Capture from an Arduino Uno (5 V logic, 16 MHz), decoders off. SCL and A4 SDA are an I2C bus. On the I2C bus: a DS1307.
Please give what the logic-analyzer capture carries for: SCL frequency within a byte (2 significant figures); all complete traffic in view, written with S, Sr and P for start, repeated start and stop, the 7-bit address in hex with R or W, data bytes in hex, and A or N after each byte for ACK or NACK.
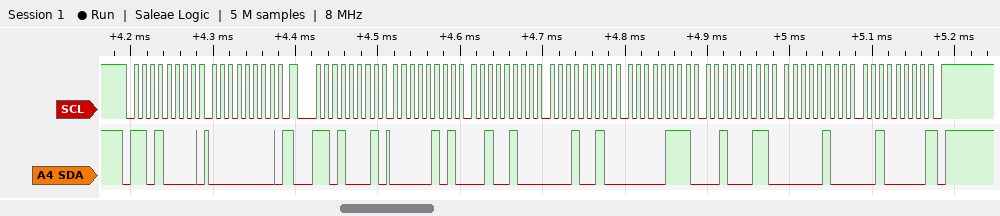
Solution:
100 kHz
S 68W A 00 A Sr 68R A 05 A 24 A 12 A 07 A 23 A 04 A 20 N P
